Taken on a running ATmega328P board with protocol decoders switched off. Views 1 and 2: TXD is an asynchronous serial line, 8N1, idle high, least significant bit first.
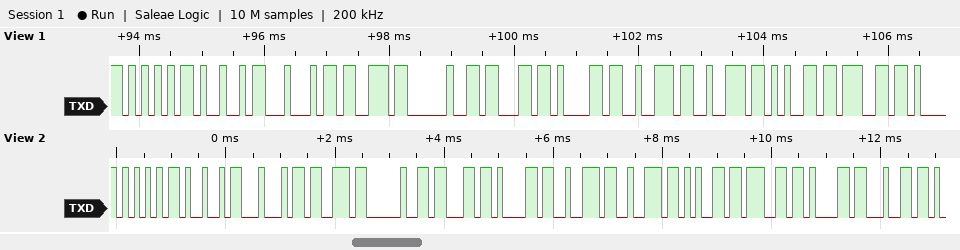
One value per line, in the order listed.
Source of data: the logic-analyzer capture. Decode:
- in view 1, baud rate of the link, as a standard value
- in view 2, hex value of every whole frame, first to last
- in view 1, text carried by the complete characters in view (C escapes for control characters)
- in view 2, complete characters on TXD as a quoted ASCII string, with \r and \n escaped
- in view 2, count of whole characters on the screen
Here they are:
9600 baud
55 49 44 73 20 63 61 72 72 65 67 61 64
"UIDs carreg"
"UIDs carregad"
13
